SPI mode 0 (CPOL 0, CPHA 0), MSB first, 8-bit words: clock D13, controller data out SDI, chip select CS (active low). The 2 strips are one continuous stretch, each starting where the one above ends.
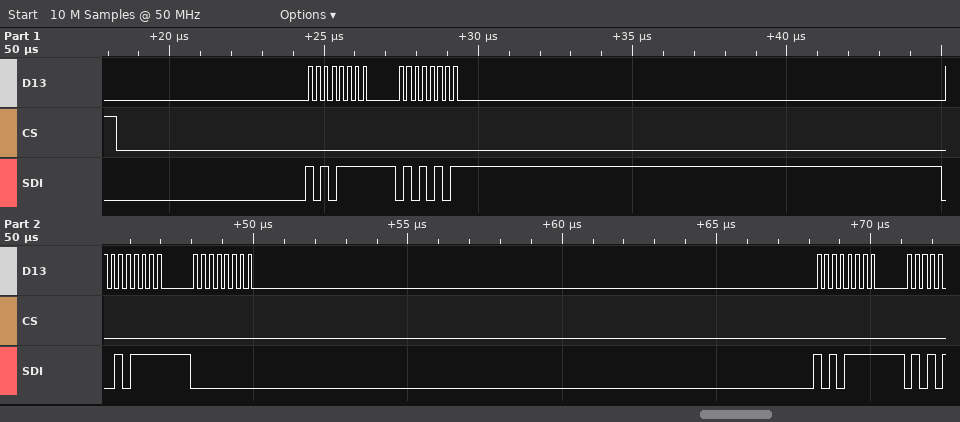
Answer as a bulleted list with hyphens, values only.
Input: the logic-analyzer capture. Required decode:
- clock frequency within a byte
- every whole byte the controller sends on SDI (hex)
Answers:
- 4 MHz
- AF 55 2F 00 AF
